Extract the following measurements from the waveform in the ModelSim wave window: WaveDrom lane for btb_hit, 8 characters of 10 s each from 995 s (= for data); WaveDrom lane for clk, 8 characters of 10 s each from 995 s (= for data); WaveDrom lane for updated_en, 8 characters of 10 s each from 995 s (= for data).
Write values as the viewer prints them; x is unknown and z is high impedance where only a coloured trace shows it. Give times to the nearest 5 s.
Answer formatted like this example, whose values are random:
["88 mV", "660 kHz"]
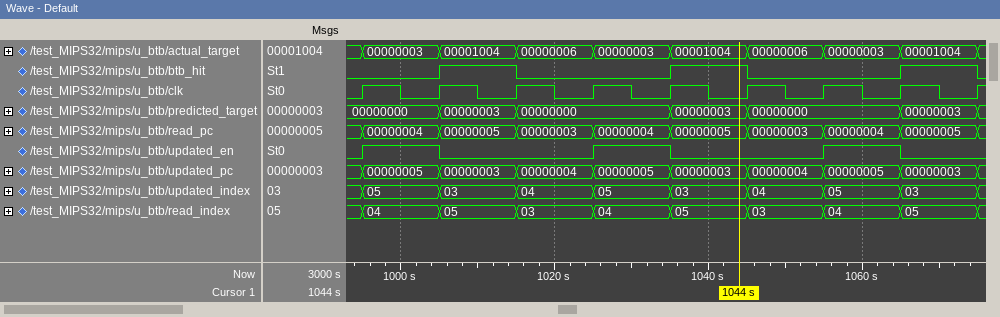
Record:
["{name: 'btb_hit', wave: '010.10.1'}", "{name: 'clk', wave: 'p.......'}", "{name: 'updated_en', wave: '10.10.10'}"]
